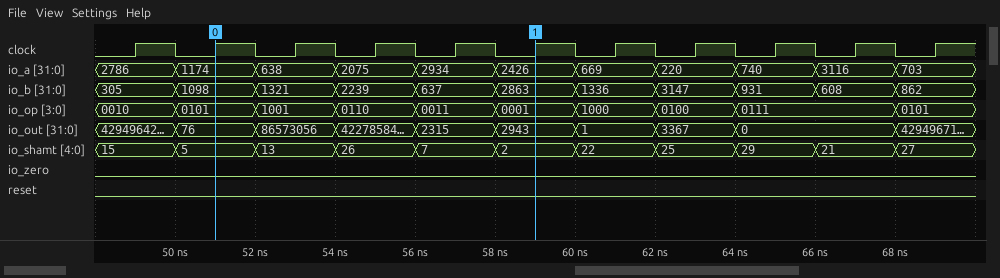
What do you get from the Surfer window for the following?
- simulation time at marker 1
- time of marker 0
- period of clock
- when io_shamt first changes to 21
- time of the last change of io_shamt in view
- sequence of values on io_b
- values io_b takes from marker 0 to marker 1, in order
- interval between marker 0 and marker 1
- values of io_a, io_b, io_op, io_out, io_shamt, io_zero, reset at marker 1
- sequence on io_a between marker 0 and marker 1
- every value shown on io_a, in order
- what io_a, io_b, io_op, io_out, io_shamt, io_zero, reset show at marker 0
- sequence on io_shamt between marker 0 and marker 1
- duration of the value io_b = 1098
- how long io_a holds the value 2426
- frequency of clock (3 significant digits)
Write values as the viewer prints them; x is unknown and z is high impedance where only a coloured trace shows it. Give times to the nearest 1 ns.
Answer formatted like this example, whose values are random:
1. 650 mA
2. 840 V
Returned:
1. 59 ns
2. 51 ns
3. 2 ns
4. 66 ns
5. 68 ns
6. 305, 1098, 1321, 2239, 637, 2863, 1336, 3147, 931, 608, 862
7. 1098, 1321, 2239, 637, 2863
8. 8 ns
9. io_a=2426, io_b=2863, io_op=0001, io_out=2943, io_shamt=2, io_zero=0, reset=0
10. 1174, 638, 2075, 2934, 2426
11. 2786, 1174, 638, 2075, 2934, 2426, 669, 220, 740, 3116, 703
12. io_a=1174, io_b=1098, io_op=0101, io_out=76, io_shamt=5, io_zero=0, reset=0
13. 5, 13, 26, 7, 2
14. 2 ns
15. 2 ns
16. 500 MHz
